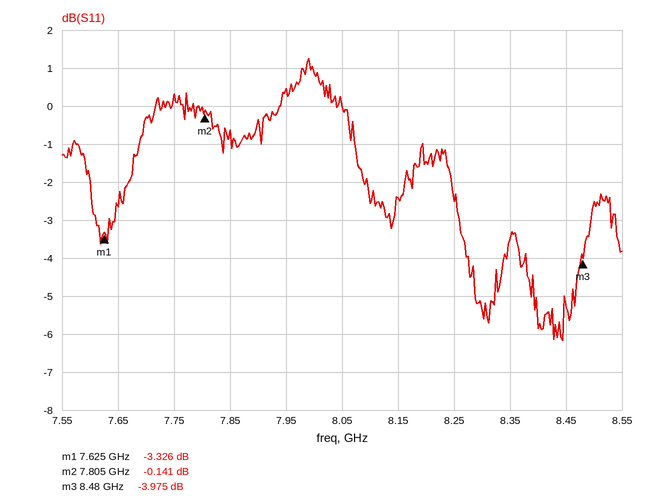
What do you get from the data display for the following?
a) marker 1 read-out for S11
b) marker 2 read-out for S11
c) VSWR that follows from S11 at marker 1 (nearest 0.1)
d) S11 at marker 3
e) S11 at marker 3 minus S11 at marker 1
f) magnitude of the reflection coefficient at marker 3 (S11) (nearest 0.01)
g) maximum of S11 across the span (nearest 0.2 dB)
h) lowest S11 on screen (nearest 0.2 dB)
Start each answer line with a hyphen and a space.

- -3.326 dB
- -0.141 dB
- 5.3
- -3.975 dB
- -0.649 dB
- 0.63
- 1.2 dB
- -6.2 dB
